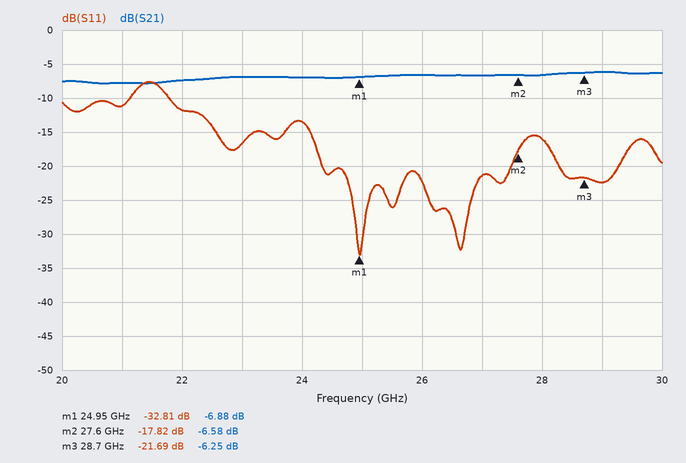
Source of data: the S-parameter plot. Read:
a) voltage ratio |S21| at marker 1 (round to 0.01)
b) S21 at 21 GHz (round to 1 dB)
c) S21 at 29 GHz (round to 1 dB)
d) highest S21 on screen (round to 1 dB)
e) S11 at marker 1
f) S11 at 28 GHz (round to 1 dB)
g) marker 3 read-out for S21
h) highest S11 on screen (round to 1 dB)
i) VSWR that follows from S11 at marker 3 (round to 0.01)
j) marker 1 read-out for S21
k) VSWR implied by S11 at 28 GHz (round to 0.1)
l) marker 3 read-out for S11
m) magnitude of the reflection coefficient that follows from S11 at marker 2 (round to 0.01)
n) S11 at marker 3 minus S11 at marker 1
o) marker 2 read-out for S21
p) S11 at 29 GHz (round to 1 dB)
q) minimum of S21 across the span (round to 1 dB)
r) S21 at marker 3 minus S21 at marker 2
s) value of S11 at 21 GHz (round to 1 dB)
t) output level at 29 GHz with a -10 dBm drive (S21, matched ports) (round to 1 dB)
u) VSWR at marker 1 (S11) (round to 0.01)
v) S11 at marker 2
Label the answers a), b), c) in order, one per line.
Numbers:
a) 0.45
b) -8 dB
c) -6 dB
d) -6 dB
e) -32.81 dB
f) -16 dB
g) -6.25 dB
h) -8 dB
i) 1.18
j) -6.88 dB
k) 1.4
l) -21.69 dB
m) 0.13
n) 11.12 dB
o) -6.58 dB
p) -22 dB
q) -8 dB
r) 0.33 dB
s) -11 dB
t) -16 dBm
u) 1.05
v) -17.82 dB
